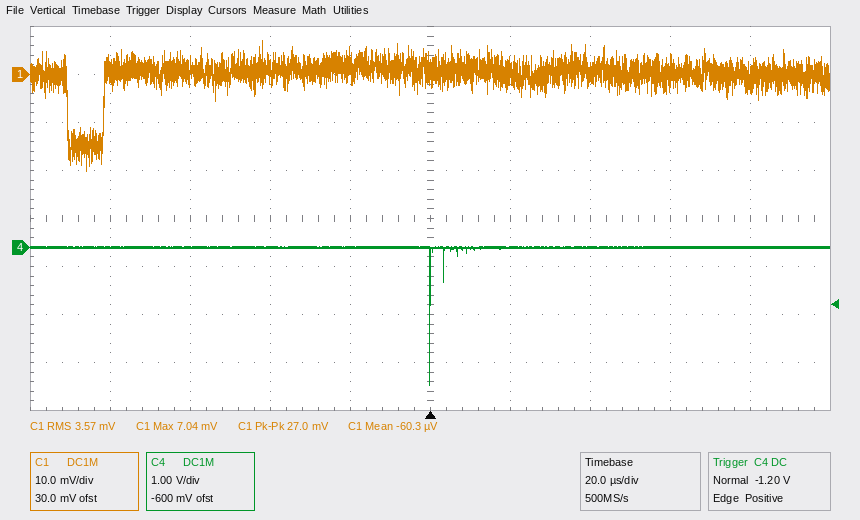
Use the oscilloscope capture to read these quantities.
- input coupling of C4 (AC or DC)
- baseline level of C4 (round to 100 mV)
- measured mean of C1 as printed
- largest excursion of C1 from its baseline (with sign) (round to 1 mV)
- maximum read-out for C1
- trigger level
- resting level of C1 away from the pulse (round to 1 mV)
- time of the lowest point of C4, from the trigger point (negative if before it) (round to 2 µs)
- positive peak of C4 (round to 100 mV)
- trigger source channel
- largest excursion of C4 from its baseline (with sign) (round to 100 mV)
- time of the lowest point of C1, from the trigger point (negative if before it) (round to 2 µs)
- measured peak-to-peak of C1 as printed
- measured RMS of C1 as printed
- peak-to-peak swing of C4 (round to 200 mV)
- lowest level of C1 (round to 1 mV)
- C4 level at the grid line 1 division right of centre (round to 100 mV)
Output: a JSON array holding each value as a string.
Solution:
["DC", "0.0 V", "-60.3 µV", "-21 mV", "7.04 mV", "-1.20 V", "1 mV", "0 µs", "0.0 V", "C4", "-2.9 V", "-86 µs", "27.0 mV", "3.57 mV", "2.8 V", "-20 mV", "0.0 V"]
